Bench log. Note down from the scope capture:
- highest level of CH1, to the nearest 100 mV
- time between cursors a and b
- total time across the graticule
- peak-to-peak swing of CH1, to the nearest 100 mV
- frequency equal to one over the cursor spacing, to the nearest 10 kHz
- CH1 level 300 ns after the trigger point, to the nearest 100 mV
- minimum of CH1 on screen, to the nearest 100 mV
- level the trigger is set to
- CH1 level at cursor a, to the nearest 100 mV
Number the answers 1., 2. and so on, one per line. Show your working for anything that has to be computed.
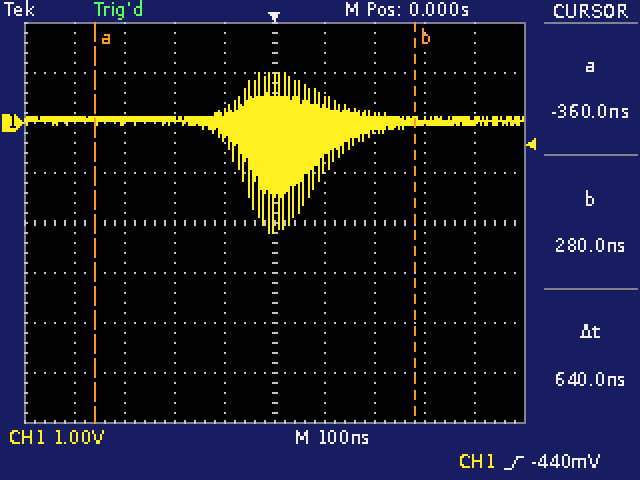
1. 1.0 V
2. 640 ns
3. 1 µs
4. 1.0 V − (-2.2 V) = 3.2 V
5. 1 / 640 ns ≈ 1.56 MHz
6. 0.0 V
7. -2.2 V
8. -440 mV
9. 100 mV
